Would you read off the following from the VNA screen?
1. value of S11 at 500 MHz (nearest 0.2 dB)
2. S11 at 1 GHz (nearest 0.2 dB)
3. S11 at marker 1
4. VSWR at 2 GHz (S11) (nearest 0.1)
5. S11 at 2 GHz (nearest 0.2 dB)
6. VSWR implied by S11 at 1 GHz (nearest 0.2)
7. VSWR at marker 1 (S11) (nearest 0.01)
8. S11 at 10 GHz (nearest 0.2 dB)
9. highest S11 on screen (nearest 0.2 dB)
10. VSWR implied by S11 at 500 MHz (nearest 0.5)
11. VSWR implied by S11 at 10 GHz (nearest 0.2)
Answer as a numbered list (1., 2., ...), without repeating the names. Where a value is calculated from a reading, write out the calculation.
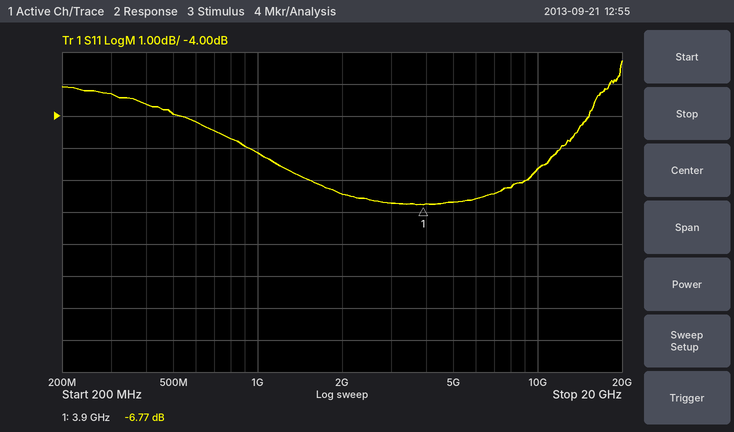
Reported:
1. -4.0 dB
2. -5.2 dB
3. -6.77 dB
4. |Γ| = 10^(-6.4/20) = 0.4786; VSWR = (1 + 0.4786)/(1 − 0.4786) ≈ 2.8
5. -6.4 dB
6. |Γ| = 10^(-5.2/20) = 0.5495; VSWR = (1 + 0.5495)/(1 − 0.5495) ≈ 3.4
7. (1 + 0.4587)/(1 − 0.4587) ≈ 2.69
8. -5.6 dB
9. -2.2 dB
10. |Γ| = 10^(-4/20) = 0.6310; VSWR = (1 + 0.6310)/(1 − 0.6310) ≈ 4.42, so 4.5 to the nearest 0.5
11. |Γ| = 10^(-5.6/20) = 0.5248; VSWR = (1 + 0.5248)/(1 − 0.5248) ≈ 3.2
